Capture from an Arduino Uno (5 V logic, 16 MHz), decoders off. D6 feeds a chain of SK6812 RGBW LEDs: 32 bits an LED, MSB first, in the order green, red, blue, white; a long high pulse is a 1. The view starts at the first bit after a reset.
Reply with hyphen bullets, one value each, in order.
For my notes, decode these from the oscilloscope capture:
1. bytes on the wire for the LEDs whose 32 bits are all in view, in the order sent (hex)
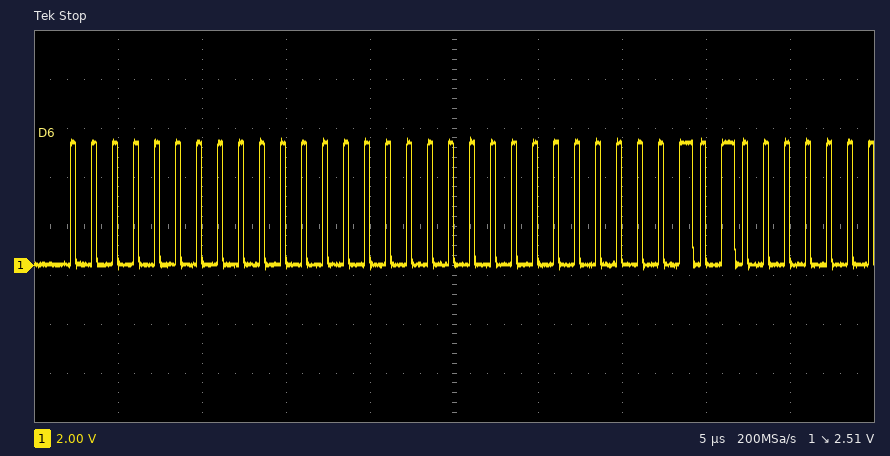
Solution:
- 00 00 00 05
